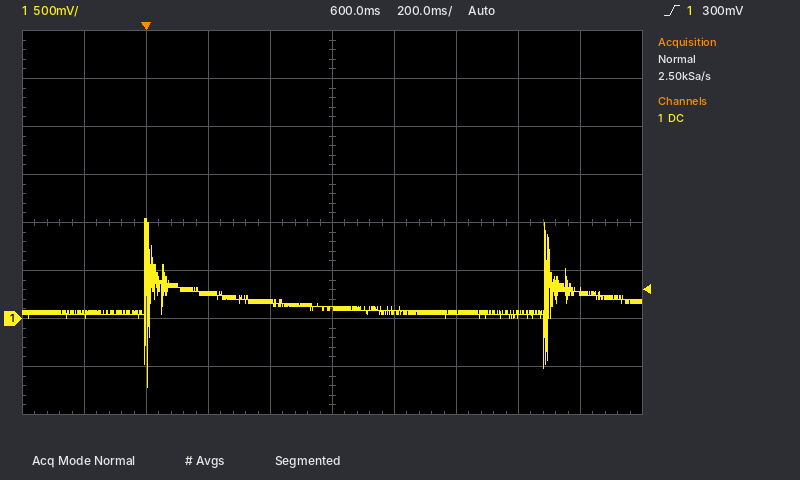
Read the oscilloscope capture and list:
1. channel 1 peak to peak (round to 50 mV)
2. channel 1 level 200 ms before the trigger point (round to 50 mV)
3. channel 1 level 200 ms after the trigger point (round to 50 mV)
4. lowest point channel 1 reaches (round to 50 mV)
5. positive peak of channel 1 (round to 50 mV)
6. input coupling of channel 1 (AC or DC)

1.75 V
50 mV
250 mV
-700 mV
1.05 V
DC
